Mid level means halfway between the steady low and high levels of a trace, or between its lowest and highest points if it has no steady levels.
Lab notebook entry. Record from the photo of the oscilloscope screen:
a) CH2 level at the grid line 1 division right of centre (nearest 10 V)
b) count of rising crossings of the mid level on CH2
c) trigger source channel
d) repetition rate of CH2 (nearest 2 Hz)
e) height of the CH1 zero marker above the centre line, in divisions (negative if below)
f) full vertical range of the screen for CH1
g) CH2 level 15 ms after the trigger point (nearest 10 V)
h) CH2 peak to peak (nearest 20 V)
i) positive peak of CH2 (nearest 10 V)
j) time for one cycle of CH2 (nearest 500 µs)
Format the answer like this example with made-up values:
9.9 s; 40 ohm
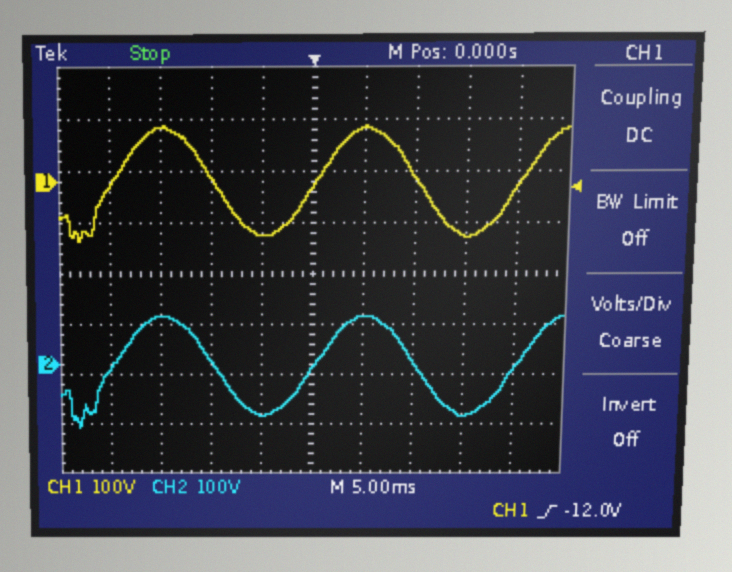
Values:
100 V; 3; CH1; 50 Hz; +1.8 div; 800 V; -100 V; 220 V; 100 V; 20.0 ms
